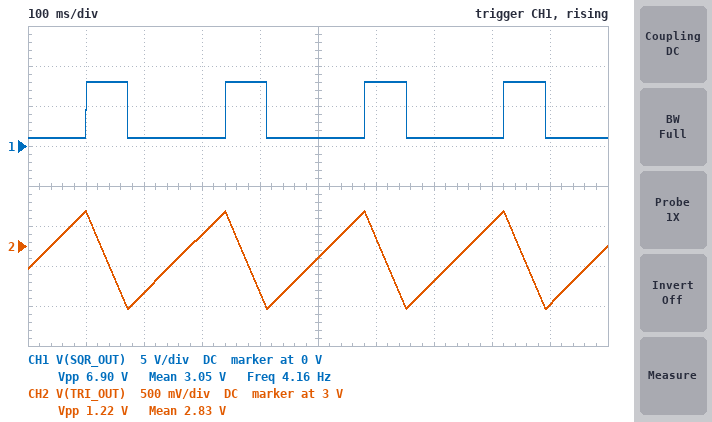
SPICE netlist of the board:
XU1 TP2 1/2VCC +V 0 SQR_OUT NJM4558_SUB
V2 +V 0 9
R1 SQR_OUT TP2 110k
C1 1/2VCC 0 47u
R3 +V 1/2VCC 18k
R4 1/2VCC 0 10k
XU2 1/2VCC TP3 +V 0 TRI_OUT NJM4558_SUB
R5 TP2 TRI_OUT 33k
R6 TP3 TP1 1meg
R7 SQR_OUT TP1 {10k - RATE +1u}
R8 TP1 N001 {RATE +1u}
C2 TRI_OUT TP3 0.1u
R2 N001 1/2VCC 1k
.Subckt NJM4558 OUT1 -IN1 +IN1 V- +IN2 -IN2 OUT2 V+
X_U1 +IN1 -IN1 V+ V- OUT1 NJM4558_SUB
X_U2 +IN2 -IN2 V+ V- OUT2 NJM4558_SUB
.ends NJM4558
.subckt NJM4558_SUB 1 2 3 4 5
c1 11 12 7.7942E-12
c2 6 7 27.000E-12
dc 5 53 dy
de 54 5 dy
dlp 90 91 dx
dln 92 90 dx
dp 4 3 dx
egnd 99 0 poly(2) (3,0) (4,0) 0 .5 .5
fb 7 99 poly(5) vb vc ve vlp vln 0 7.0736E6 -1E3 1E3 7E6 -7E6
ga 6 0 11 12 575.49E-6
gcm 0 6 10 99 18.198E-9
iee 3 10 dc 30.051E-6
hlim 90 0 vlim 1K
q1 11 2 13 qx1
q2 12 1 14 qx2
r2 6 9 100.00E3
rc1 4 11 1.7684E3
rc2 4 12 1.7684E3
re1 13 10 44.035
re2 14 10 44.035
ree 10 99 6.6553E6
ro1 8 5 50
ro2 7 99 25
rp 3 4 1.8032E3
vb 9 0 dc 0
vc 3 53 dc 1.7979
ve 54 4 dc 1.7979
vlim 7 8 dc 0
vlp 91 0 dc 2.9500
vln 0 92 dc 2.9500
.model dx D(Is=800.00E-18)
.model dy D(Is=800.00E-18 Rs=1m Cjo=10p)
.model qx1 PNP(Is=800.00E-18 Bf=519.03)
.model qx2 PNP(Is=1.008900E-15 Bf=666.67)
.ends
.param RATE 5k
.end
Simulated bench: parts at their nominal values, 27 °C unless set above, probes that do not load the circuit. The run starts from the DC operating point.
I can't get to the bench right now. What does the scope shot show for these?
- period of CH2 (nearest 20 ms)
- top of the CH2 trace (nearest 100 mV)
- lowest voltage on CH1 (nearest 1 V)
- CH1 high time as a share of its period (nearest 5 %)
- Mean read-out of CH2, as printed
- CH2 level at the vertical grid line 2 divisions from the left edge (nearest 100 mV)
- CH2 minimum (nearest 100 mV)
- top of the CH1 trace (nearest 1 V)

240 ms
3.4 V
1 V
30 %
2.83 V
2.4 V
2.2 V
8 V
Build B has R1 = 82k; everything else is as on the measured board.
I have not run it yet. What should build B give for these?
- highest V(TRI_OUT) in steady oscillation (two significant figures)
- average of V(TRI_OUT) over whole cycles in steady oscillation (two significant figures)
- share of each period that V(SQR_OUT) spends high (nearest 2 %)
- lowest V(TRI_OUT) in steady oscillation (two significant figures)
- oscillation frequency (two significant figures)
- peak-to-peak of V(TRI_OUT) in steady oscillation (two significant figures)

3.5 V
2.7 V
30 %
1.9 V
3.2 Hz
1.6 V
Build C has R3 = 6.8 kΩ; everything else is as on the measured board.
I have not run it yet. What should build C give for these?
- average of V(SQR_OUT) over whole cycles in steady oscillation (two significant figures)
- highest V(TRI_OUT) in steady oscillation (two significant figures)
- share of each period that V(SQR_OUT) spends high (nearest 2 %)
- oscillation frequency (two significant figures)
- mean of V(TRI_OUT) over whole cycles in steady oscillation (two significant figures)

5.3 V
6.2 V
62 %
4.7 Hz
5.6 V
